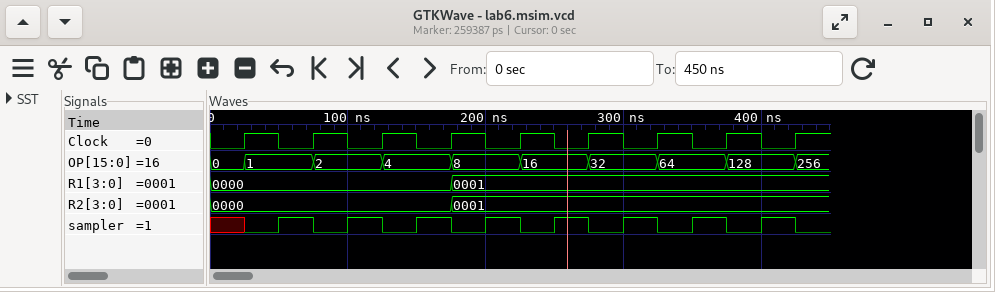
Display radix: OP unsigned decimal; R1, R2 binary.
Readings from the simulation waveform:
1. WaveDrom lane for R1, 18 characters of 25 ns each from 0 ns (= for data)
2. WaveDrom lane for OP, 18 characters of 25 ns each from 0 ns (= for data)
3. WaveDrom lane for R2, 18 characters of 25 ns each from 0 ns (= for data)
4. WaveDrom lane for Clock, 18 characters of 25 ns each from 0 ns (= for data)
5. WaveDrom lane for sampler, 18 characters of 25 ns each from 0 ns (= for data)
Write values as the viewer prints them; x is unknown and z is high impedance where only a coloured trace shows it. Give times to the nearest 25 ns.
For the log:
{name: 'R1', wave: '=......=..........', data: '0000 0001'}
{name: 'OP', wave: '==.=.=.=.=.=.=.=.=', data: '0 1 2 4 8 16 32 64 128 256'}
{name: 'R2', wave: '=......=..........', data: '0000 0001'}
{name: 'Clock', wave: '010101010101010101'}
{name: 'sampler', wave: 'x01010101010101010'}
